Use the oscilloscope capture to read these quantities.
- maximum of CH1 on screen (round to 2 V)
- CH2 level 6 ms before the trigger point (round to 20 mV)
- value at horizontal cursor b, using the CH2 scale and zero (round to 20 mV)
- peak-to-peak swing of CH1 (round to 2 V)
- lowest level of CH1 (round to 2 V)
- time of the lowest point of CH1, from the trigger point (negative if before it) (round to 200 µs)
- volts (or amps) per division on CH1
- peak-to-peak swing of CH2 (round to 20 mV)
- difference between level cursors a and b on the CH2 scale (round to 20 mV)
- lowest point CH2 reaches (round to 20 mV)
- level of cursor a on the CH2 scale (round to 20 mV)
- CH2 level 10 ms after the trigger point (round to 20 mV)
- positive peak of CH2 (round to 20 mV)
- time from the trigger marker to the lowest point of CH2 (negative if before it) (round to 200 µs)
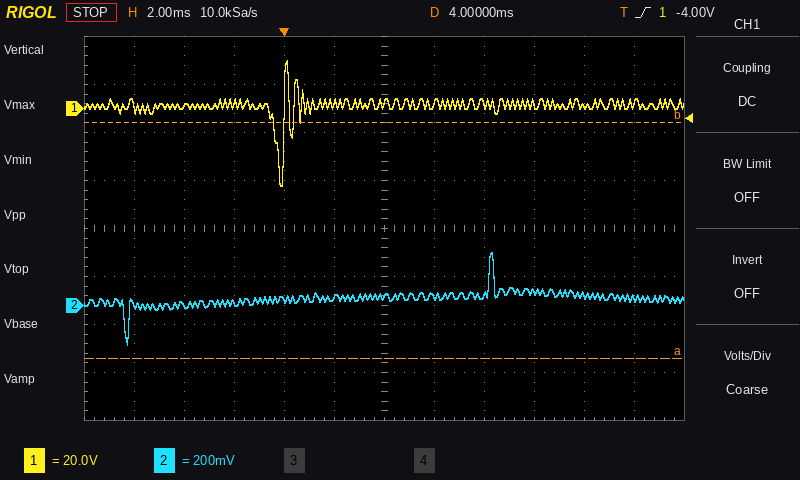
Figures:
20 V
0 mV
760 mV
52 V
-32 V
-200 µs
20 V
380 mV
980 mV
-160 mV
-220 mV
60 mV
220 mV
-6.2 ms
